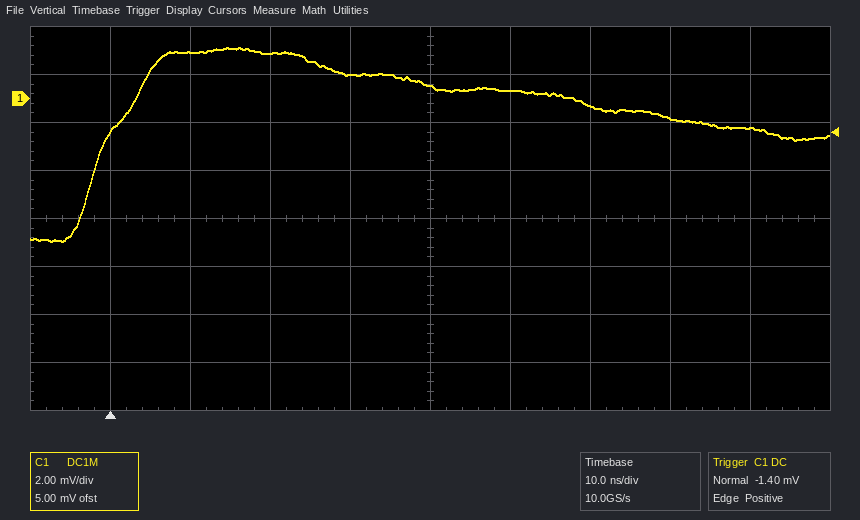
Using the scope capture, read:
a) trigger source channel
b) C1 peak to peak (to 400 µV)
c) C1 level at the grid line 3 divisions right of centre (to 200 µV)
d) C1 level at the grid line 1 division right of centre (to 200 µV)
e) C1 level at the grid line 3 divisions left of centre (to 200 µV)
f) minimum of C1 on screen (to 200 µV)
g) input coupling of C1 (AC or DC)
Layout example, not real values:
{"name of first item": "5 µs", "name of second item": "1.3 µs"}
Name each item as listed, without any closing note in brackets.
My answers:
{"trigger source channel": "C1", "C1 peak to peak": "8.0 mV", "C1 level at the grid line 3 divisions right of centre": "-800 µV", "C1 level at the grid line 1 division right of centre": "400 µV", "C1 level at the grid line 3 divisions left of centre": "2.0 mV", "minimum of C1 on screen": "-6.0 mV", "input coupling of C1": "DC"}
